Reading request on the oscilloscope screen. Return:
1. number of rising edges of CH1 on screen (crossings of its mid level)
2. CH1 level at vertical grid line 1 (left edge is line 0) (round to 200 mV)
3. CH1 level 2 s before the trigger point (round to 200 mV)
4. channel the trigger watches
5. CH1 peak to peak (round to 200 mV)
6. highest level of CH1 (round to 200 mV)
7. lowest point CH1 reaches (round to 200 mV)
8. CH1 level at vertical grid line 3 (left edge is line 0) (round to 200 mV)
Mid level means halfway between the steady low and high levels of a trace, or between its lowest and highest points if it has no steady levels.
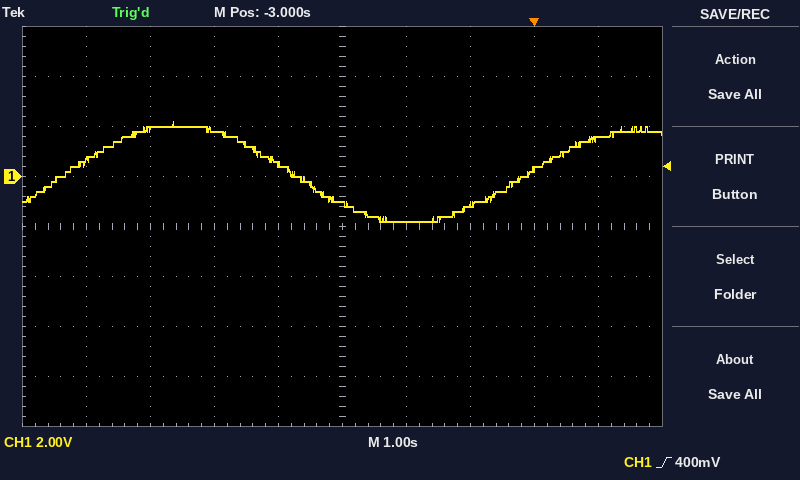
2
600 mV
-1.8 V
CH1
4.0 V
2.2 V
-1.8 V
1.8 V
